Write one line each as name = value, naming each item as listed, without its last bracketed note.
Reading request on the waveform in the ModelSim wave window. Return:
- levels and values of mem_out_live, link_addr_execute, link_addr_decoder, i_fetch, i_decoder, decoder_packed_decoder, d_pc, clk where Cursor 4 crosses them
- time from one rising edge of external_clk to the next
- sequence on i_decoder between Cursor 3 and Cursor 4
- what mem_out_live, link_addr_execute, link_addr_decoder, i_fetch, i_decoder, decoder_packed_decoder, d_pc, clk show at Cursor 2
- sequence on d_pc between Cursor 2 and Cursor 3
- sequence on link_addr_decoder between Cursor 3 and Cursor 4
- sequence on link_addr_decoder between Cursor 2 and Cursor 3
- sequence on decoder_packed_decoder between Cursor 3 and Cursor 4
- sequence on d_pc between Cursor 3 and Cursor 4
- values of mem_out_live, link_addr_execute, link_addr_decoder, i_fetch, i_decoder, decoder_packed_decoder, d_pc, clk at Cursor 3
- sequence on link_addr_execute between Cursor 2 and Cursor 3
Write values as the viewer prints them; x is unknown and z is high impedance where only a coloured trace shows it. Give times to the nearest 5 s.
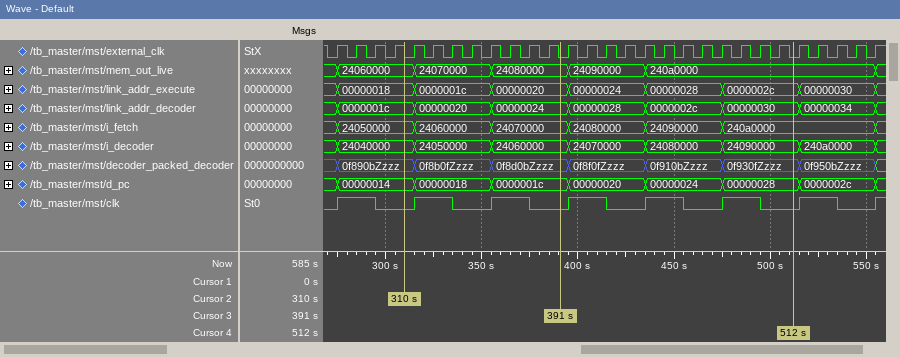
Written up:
levels and values of mem_out_live, link_addr_execute, link_addr_decoder, i_fetch, i_decoder, decoder_packed_decoder, d_pc, clk where Cursor 4 crosses them = mem_out_live=240a0000, link_addr_execute=0000002c, link_addr_decoder=00000030, i_fetch=240a0000, i_decoder=24090000, decoder_packed_decoder=0f930fZzzz, d_pc=00000028, clk=0
time from one rising edge of external_clk to the next = 10 s
sequence on i_decoder between Cursor 3 and Cursor 4 = 24060000, 24070000, 24080000, 24090000
what mem_out_live, link_addr_execute, link_addr_decoder, i_fetch, i_decoder, decoder_packed_decoder, d_pc, clk show at Cursor 2 = mem_out_live=24060000, link_addr_execute=00000018, link_addr_decoder=0000001c, i_fetch=24050000, i_decoder=24040000, decoder_packed_decoder=0f890bZzzz, d_pc=00000014, clk=0
sequence on d_pc between Cursor 2 and Cursor 3 = 00000014, 00000018, 0000001c
sequence on link_addr_decoder between Cursor 3 and Cursor 4 = 00000024, 00000028, 0000002c, 00000030
sequence on link_addr_decoder between Cursor 2 and Cursor 3 = 0000001c, 00000020, 00000024
sequence on decoder_packed_decoder between Cursor 3 and Cursor 4 = 0f8d0bZzzz, 0f8f0fZzzz, 0f910bZzzz, 0f930fZzzz
sequence on d_pc between Cursor 3 and Cursor 4 = 0000001c, 00000020, 00000024, 00000028
values of mem_out_live, link_addr_execute, link_addr_decoder, i_fetch, i_decoder, decoder_packed_decoder, d_pc, clk at Cursor 3 = mem_out_live=24080000, link_addr_execute=00000020, link_addr_decoder=00000024, i_fetch=24070000, i_decoder=24060000, decoder_packed_decoder=0f8d0bZzzz, d_pc=0000001c, clk=0
sequence on link_addr_execute between Cursor 2 and Cursor 3 = 00000018, 0000001c, 00000020
